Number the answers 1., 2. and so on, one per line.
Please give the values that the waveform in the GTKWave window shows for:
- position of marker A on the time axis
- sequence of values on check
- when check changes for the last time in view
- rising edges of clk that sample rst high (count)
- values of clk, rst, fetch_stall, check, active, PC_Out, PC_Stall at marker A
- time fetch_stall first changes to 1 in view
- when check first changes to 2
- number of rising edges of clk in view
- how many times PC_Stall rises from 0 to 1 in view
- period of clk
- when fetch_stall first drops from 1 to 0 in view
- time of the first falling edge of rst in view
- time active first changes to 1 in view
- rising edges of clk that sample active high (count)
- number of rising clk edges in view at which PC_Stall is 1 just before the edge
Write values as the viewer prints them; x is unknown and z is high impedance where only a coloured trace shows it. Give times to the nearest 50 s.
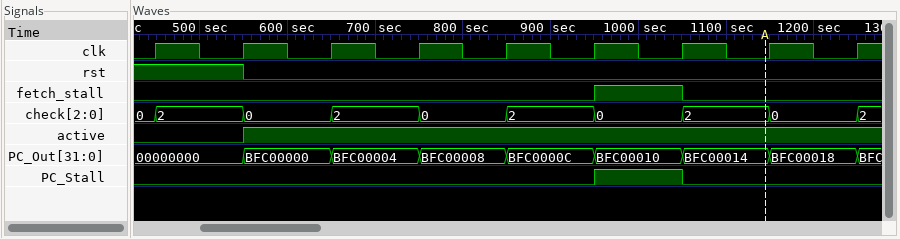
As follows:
1. 1150 s
2. 0, 2, 0, 2, 0, 2, 0, 2, 0, 2
3. 1250 s
4. 2
5. clk=0, rst=0, fetch_stall=0, check=2, active=1, PC_Out=BFC00014, PC_Stall=0
6. 950 s
7. 450 s
8. 9
9. 1
10. 100 s
11. 1050 s
12. 550 s
13. 550 s
14. 7
15. 1
